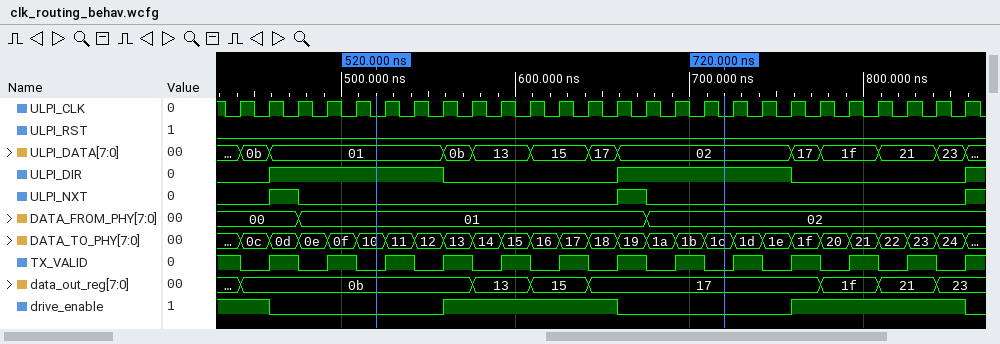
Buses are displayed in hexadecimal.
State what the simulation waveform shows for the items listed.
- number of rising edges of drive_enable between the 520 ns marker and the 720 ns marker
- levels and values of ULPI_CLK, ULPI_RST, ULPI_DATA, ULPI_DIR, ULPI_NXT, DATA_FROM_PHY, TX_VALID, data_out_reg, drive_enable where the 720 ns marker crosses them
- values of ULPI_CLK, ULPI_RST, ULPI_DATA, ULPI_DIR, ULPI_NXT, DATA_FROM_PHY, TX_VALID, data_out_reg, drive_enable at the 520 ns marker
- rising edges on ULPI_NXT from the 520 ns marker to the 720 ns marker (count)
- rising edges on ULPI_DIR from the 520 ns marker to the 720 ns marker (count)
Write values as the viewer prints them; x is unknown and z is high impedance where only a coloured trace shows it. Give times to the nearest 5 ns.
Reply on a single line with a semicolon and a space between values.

1; ULPI_CLK=0, ULPI_RST=0, ULPI_DATA=02, ULPI_DIR=1, ULPI_NXT=0, DATA_FROM_PHY=02, TX_VALID=0, data_out_reg=17, drive_enable=0; ULPI_CLK=0, ULPI_RST=0, ULPI_DATA=01, ULPI_DIR=1, ULPI_NXT=0, DATA_FROM_PHY=01, TX_VALID=0, data_out_reg=0b, drive_enable=0; 1; 1
